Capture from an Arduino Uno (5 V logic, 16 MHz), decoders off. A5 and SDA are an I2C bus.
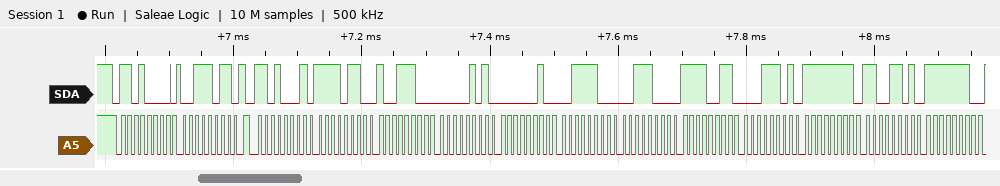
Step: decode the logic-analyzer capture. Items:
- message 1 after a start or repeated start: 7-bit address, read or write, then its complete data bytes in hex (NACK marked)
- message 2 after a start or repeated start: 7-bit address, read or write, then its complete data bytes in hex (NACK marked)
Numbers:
0x68 write: 3B
0x68 read: F6 9C 05 02 3C 38 F3 1D FF CD FE
